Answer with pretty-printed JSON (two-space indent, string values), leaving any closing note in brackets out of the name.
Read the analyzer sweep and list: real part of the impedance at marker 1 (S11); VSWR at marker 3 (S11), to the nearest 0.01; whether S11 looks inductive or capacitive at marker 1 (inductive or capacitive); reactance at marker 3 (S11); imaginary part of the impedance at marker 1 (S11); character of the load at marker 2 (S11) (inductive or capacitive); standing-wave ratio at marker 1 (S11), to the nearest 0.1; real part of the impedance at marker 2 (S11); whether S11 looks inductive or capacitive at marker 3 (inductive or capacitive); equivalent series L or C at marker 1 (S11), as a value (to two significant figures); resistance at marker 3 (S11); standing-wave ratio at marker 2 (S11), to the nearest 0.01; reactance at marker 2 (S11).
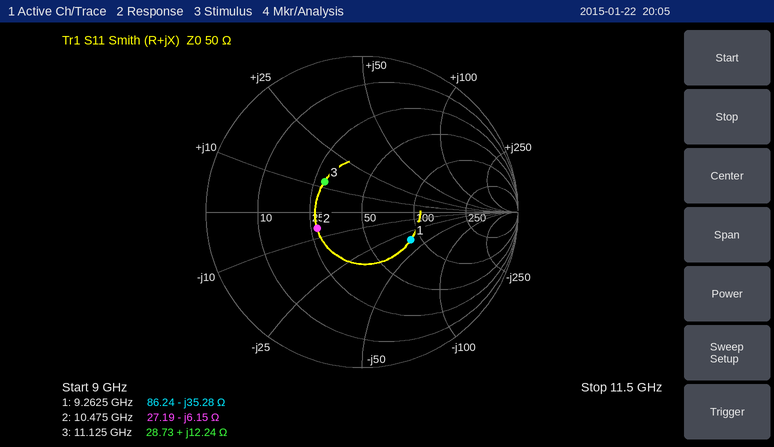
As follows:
{
  "real part of the impedance at marker 1": "86.24 Ω",
  "VSWR at marker 3 (S11), to the nearest 0.01": "1.89",
  "whether S11 looks inductive or capacitive at marker 1": "capacitive",
  "reactance at marker 3": "+12.24 Ω",
  "imaginary part of the impedance at marker 1": "-35.28 Ω",
  "character of the load at marker 2 (S11)": "capacitive",
  "standing-wave ratio at marker 1 (S11), to the nearest 0.1": "2.1",
  "real part of the impedance at marker 2": "27.19 Ω",
  "whether S11 looks inductive or capacitive at marker 3": "inductive",
  "equivalent series L or C at marker 1 (S11), as a value": "490 fF",
  "resistance at marker 3": "28.73 Ω",
  "standing-wave ratio at marker 2 (S11), to the nearest 0.01": "1.88",
  "reactance at marker 2": "-6.15 Ω"
}
